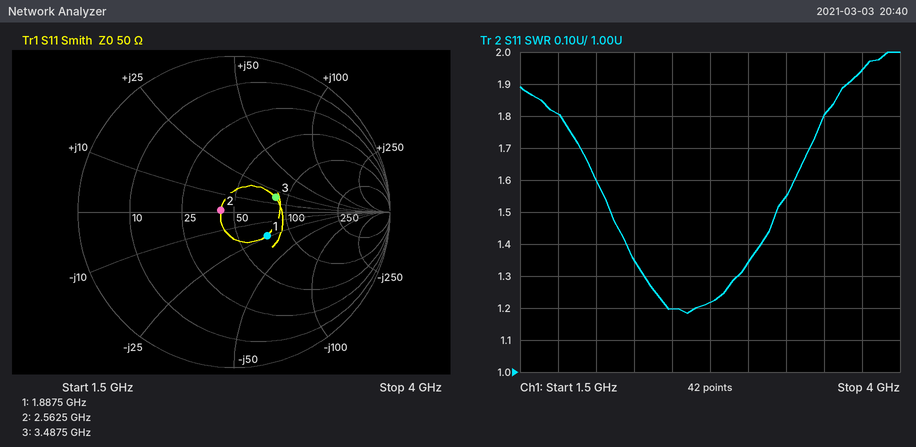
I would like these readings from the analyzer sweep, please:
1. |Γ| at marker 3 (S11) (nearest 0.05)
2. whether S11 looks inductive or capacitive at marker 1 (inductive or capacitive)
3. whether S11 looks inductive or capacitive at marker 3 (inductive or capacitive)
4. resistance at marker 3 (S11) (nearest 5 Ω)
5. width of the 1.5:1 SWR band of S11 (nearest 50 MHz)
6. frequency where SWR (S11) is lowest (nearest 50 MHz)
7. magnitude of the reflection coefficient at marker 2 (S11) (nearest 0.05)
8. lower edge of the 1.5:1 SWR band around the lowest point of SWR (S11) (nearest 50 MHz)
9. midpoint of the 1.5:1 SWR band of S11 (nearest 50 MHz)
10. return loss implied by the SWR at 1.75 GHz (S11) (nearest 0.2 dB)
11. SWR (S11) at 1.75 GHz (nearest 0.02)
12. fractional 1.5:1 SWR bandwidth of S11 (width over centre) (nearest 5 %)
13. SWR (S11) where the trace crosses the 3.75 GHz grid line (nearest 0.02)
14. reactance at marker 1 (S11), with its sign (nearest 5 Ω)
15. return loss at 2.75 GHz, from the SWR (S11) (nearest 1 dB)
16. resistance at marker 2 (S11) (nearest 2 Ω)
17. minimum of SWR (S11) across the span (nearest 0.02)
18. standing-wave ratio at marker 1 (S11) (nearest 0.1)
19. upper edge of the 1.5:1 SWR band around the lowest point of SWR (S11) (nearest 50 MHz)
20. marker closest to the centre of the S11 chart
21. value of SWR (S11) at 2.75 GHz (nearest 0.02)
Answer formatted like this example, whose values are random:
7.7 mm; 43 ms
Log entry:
0.30; capacitive; inductive; 85 Ω; 1.10 GHz; 2.60 GHz; 0.10; 2.10 GHz; 2.65 GHz; 10.8 dB; 1.80; 40 %; 1.94; -25 Ω; 20 dB; 42 Ω; 1.18; 1.7; 3.20 GHz; marker 2; 1.22
